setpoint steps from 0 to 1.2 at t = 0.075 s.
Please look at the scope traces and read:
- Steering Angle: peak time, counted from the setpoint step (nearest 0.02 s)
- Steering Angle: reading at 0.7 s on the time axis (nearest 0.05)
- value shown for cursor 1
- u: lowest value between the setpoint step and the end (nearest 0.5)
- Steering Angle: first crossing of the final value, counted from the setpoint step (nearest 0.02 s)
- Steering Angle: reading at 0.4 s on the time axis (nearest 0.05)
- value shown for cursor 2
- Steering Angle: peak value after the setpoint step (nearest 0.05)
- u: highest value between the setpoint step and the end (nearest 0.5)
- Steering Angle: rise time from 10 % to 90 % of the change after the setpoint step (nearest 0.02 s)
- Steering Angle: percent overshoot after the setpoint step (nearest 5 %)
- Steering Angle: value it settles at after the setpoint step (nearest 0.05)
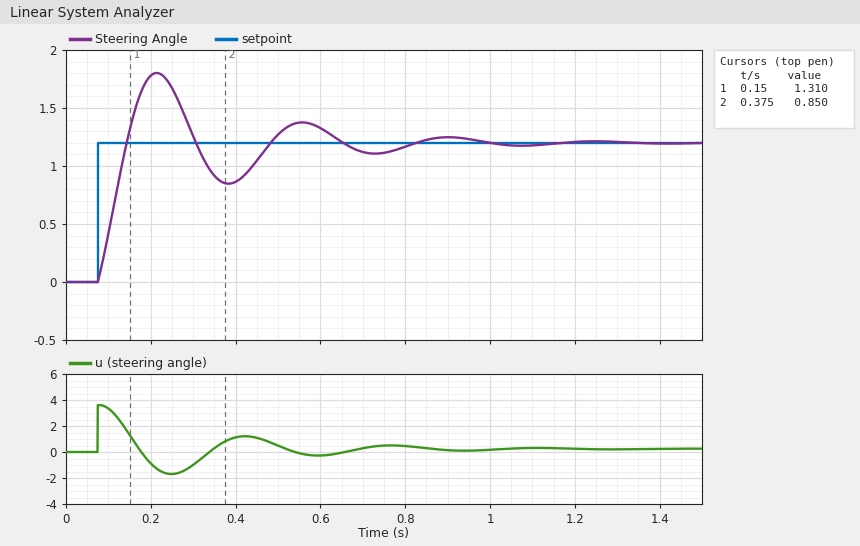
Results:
0.14 s
1.10
1.310
-1.5
0.06 s
0.85
0.850
1.80
3.5
0.06 s
50 %
1.20
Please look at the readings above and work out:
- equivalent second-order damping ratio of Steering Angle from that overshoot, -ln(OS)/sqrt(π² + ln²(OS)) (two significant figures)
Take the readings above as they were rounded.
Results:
0.22
